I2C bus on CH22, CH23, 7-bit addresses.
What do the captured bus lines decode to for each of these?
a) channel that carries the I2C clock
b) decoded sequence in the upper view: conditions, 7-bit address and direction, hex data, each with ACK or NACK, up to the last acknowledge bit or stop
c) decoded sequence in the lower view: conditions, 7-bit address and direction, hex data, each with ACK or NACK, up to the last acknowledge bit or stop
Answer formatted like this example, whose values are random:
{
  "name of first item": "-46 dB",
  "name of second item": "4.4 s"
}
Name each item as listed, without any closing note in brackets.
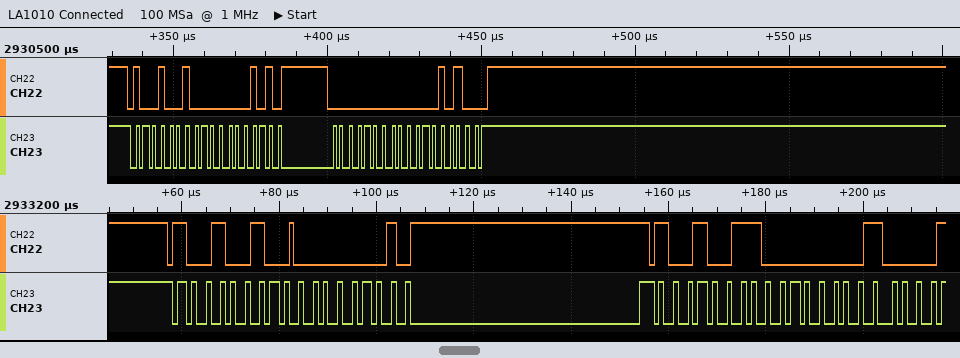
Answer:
{
  "channel that carries the I2C clock": "CH23",
  "decoded sequence in the upper view: conditions, 7-bit address and direction, hex data, each with ACK or NACK, up to the last acknowledge bit or stop": "start, address 49 write ACK, 05 ACK, 00 ACK, 0A ACK, stop",
  "decoded sequence in the lower view: conditions, 7-bit address and direction, hex data, each with ACK or NACK, up to the last acknowledge bit or stop": "start, address 49 write ACK, 01 ACK, repeated start, address 49 read ACK, 01 ACK"
}
